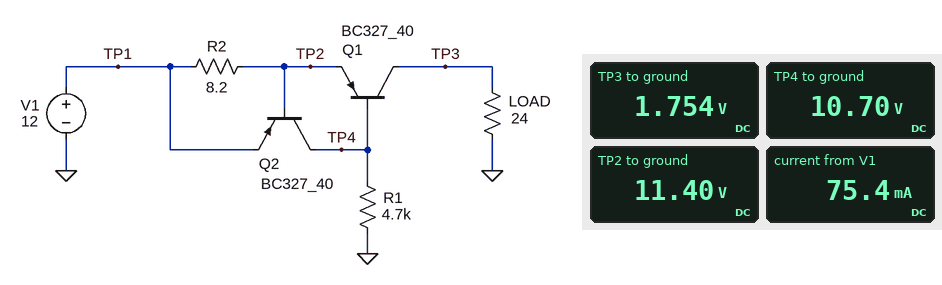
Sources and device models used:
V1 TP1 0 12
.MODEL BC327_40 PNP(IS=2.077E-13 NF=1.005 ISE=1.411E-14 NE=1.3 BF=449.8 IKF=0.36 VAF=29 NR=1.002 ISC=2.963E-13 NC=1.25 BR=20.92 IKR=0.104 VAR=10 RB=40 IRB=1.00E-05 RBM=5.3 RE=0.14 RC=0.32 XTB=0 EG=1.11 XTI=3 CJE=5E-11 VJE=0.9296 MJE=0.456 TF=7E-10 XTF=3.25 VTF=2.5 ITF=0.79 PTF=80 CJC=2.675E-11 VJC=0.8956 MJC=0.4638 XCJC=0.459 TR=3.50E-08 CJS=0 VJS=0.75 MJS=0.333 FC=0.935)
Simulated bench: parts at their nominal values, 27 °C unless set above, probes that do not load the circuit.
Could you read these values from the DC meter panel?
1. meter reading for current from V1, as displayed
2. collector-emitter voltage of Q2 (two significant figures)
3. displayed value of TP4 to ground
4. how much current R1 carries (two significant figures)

75.4 mA
-1.3 V
10.70 V
2.3 mA
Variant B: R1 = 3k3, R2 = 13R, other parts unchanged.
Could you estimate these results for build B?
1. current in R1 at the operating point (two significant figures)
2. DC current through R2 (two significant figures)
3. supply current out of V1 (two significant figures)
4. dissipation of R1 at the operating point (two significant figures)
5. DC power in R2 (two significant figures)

3.2 mA
47 mA
50 mA
35 mW
29 mW
